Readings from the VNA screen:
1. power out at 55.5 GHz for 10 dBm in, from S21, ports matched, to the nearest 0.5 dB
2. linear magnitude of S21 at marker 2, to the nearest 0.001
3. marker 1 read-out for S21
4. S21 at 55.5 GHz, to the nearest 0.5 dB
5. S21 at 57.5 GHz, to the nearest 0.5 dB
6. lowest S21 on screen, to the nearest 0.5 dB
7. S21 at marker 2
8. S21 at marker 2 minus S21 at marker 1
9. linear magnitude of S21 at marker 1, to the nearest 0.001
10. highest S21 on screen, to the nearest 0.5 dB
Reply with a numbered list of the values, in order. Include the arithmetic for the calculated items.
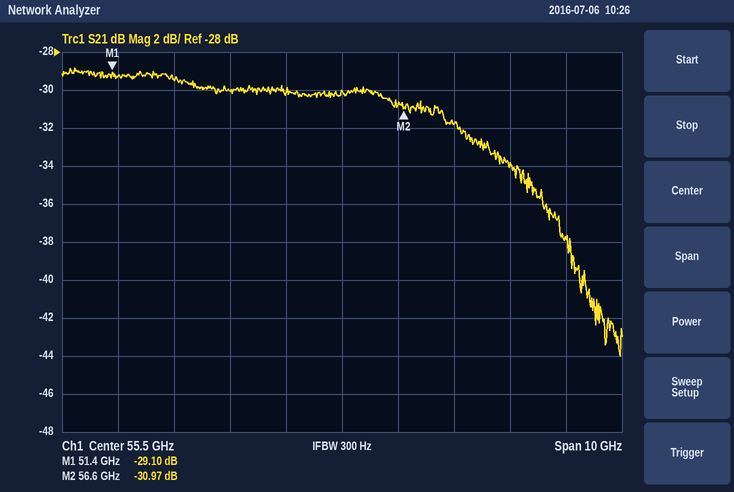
1. 10 dBm + (-30.0 dB) = -20.0 dBm
2. 10^(-30.97/20) ≈ 0.028
3. -29.10 dB
4. -30.0 dB
5. -32.0 dB
6. -44.0 dB
7. -30.97 dB
8. -30.97 − (-29.1) = -1.87 dB
9. 10^(-29.1/20) ≈ 0.035
10. -29.0 dB
